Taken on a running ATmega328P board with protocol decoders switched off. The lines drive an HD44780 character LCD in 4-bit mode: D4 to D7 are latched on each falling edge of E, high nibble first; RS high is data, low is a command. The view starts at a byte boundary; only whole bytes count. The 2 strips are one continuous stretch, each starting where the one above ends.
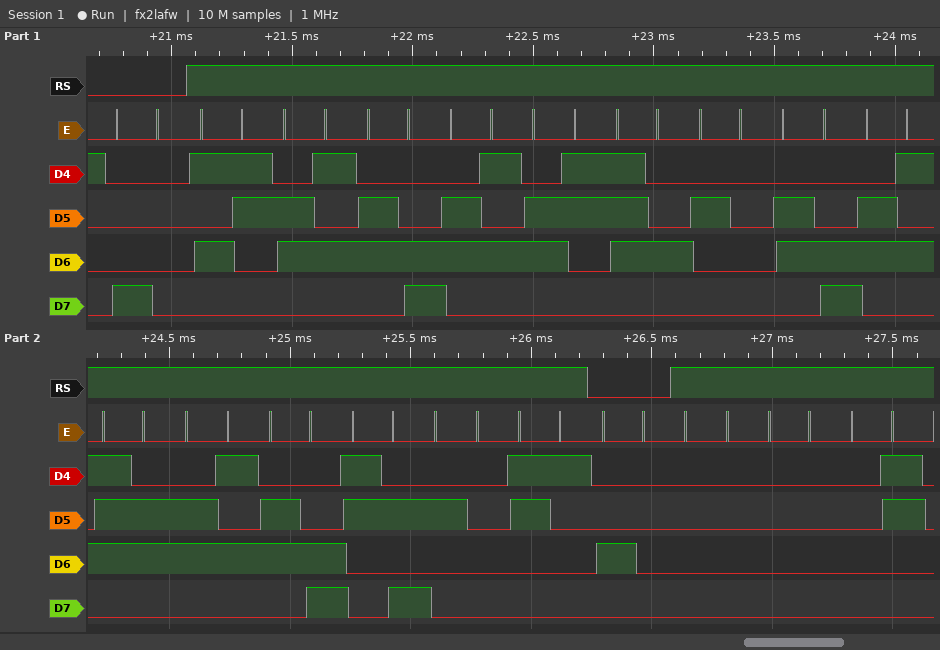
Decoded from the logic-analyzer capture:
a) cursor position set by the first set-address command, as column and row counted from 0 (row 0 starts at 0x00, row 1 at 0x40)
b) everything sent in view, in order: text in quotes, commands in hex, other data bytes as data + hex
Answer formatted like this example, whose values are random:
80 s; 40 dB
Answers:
column 0, row 0; 0x80 "Select level: 1" 0x40 data 00 00 03
